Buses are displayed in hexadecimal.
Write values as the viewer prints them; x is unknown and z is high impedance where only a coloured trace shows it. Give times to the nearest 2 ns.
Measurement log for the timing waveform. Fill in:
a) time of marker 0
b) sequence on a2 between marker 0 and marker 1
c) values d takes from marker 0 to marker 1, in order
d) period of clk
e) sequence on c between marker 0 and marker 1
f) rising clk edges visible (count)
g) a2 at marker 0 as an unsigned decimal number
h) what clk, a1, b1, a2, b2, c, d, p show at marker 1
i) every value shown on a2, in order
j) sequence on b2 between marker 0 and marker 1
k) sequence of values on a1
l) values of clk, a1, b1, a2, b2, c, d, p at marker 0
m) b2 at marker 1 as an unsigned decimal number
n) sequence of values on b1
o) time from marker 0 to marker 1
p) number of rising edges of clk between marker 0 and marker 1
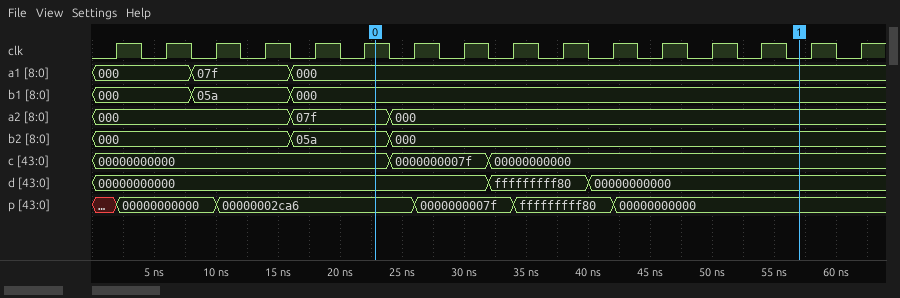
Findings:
22 ns
07f, 000
00000000000, fffffffff80, 00000000000
4 ns
00000000000, 0000000007f, 00000000000
16
127
clk=0, a1=000, b1=000, a2=000, b2=000, c=00000000000, d=00000000000, p=00000000000
000, 07f, 000
05a, 000
000, 07f, 000
clk=1, a1=000, b1=000, a2=07f, b2=05a, c=00000000000, d=00000000000, p=00000002ca6
0
000, 05a, 000
34 ns
8
